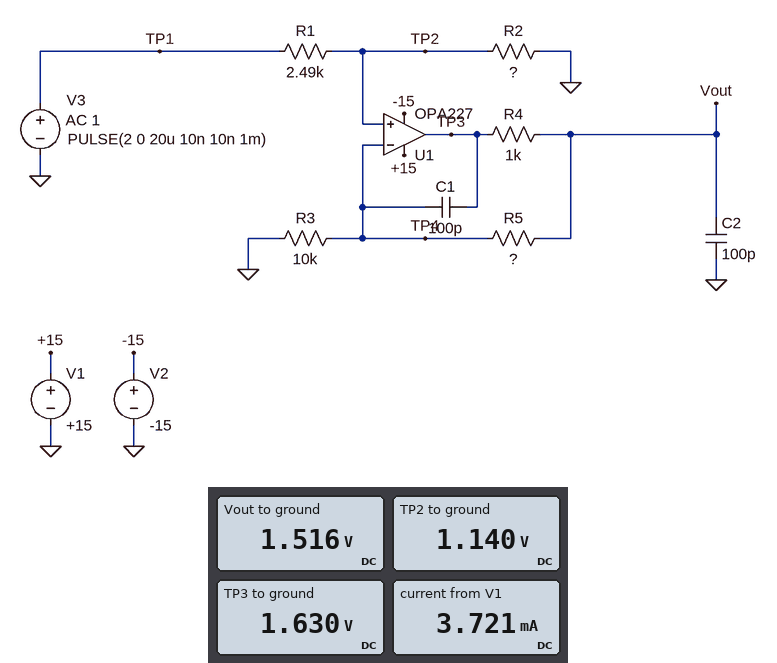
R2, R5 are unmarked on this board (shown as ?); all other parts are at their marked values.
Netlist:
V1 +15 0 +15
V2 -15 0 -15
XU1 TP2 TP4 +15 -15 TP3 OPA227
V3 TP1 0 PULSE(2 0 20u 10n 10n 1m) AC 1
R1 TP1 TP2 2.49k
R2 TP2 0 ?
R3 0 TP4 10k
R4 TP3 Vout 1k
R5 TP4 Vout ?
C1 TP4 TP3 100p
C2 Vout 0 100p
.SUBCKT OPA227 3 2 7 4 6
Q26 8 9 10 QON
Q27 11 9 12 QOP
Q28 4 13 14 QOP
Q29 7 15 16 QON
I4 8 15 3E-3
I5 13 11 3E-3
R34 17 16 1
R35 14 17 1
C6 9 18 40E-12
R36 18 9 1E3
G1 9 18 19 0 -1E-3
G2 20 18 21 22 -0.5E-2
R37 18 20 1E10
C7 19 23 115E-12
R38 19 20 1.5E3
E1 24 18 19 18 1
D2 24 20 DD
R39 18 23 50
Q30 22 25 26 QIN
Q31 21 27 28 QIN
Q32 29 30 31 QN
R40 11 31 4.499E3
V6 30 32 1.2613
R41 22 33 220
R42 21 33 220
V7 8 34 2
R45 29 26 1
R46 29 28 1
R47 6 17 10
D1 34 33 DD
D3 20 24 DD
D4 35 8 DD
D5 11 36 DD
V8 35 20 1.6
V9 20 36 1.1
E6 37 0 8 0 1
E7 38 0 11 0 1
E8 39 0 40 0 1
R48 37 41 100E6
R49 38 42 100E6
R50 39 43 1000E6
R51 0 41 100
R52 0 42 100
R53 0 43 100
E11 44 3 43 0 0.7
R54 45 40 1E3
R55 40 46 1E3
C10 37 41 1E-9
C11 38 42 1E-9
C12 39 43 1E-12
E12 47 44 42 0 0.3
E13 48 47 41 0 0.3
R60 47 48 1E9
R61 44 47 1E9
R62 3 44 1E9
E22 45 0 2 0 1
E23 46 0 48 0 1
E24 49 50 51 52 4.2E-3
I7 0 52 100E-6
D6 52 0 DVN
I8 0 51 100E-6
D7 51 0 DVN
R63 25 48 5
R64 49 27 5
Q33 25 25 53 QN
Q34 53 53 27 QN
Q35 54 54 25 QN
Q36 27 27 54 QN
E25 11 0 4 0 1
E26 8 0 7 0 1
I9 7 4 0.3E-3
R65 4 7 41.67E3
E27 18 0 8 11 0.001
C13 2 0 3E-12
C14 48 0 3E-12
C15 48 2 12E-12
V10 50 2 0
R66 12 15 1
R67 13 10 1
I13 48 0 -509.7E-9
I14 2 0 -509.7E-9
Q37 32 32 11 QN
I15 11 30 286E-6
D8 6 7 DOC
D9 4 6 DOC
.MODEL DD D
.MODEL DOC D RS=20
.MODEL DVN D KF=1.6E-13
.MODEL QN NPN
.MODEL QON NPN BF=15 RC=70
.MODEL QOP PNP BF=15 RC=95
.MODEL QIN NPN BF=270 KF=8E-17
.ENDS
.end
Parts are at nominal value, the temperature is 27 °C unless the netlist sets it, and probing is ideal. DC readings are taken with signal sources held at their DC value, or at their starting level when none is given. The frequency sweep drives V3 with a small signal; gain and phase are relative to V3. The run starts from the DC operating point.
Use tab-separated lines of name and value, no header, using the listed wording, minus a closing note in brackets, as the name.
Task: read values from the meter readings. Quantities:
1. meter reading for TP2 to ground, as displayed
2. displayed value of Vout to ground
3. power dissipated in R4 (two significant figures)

meter reading for TP2 to ground, as displayed	1.140 V
displayed value of Vout to ground	1.516 V
power dissipated in R4	13 µW
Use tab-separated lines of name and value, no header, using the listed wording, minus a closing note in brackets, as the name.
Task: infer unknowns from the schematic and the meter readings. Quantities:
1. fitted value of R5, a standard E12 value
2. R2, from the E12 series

fitted value of R5, a standard E12 value	3.3 kΩ
R2, from the E12 series	3.3 kΩ
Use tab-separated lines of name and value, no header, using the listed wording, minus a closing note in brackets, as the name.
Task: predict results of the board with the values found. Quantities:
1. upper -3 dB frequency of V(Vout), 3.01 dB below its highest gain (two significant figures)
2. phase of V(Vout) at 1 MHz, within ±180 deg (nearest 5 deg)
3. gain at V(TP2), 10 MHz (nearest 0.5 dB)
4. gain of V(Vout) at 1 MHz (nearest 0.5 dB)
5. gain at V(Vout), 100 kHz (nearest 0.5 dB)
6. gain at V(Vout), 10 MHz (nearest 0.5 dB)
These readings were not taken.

upper -3 dB frequency of V(Vout), 3.01 dB below its highest gain	1.9 MHz
phase of V(Vout) at 1 MHz, within ±180 deg	-45 deg
gain at V(TP2), 10 MHz	-9.0 dB
gain of V(Vout) at 1 MHz	-3.5 dB
gain at V(Vout), 100 kHz	-2.5 dB
gain at V(Vout), 10 MHz	-33.0 dB
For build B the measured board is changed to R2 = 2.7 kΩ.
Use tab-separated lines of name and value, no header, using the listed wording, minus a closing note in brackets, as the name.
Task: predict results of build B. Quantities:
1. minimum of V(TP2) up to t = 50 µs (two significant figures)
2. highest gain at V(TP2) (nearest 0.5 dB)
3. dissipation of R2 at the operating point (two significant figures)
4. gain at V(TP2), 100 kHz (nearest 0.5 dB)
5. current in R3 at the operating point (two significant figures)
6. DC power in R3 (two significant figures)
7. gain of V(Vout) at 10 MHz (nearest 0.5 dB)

minimum of V(TP2) up to t = 50 µs	-26 mV
highest gain at V(TP2)	-3.0 dB
dissipation of R2 at the operating point	400 µW
gain at V(TP2), 100 kHz	-5.5 dB
current in R3 at the operating point	100 µA
DC power in R3	110 µW
gain of V(Vout) at 10 MHz	-33.5 dB
